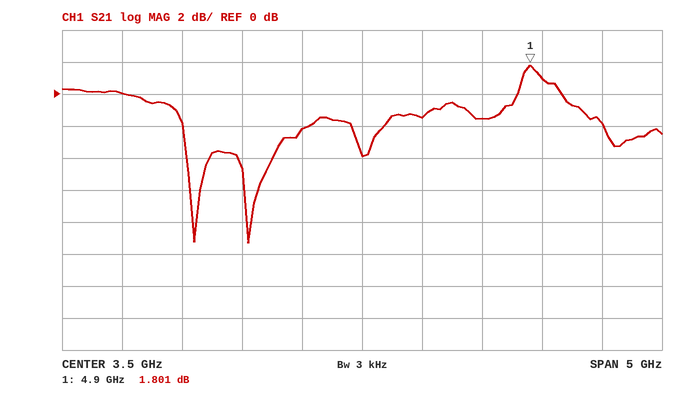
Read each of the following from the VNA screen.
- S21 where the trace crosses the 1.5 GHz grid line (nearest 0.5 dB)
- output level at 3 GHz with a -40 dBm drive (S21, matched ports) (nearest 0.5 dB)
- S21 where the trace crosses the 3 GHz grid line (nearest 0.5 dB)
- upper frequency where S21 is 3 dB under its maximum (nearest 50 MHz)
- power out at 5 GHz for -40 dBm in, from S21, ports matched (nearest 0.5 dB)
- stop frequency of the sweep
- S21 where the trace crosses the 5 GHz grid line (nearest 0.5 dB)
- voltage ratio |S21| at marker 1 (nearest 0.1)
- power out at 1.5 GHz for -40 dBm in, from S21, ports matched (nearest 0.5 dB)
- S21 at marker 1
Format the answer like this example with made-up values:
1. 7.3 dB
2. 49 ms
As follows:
1. 0.0 dB
2. -42.0 dBm
3. -2.0 dB
4. 5.35 GHz
5. -39.0 dBm
6. 6 GHz
7. 1.0 dB
8. 1.2
9. -40.0 dBm
10. 1.801 dB
